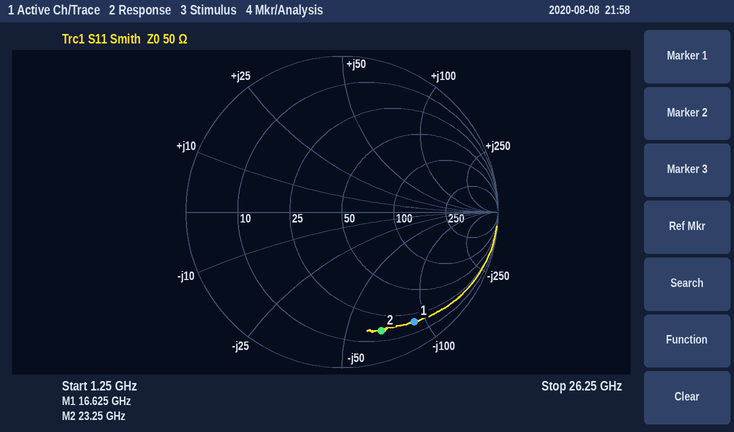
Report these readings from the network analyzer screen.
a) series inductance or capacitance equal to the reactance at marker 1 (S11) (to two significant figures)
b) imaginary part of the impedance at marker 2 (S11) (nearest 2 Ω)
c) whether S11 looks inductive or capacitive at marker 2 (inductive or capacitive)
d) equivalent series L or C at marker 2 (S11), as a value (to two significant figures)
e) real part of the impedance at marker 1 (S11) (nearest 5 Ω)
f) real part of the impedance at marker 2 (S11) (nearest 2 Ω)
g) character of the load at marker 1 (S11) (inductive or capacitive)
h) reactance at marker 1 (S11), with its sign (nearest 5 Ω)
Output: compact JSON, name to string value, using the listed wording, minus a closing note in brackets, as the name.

{"series inductance or capacitance equal to the reactance at marker 1 (S11)": "110 fF", "imaginary part of the impedance at marker 2 (S11)": "-66 Ω", "whether S11 looks inductive or capacitive at marker 2": "capacitive", "equivalent series L or C at marker 2 (S11), as a value": "100 fF", "real part of the impedance at marker 1 (S11)": "20 Ω", "real part of the impedance at marker 2 (S11)": "16 Ω", "character of the load at marker 1 (S11)": "capacitive", "reactance at marker 1 (S11), with its sign": "-90 Ω"}
